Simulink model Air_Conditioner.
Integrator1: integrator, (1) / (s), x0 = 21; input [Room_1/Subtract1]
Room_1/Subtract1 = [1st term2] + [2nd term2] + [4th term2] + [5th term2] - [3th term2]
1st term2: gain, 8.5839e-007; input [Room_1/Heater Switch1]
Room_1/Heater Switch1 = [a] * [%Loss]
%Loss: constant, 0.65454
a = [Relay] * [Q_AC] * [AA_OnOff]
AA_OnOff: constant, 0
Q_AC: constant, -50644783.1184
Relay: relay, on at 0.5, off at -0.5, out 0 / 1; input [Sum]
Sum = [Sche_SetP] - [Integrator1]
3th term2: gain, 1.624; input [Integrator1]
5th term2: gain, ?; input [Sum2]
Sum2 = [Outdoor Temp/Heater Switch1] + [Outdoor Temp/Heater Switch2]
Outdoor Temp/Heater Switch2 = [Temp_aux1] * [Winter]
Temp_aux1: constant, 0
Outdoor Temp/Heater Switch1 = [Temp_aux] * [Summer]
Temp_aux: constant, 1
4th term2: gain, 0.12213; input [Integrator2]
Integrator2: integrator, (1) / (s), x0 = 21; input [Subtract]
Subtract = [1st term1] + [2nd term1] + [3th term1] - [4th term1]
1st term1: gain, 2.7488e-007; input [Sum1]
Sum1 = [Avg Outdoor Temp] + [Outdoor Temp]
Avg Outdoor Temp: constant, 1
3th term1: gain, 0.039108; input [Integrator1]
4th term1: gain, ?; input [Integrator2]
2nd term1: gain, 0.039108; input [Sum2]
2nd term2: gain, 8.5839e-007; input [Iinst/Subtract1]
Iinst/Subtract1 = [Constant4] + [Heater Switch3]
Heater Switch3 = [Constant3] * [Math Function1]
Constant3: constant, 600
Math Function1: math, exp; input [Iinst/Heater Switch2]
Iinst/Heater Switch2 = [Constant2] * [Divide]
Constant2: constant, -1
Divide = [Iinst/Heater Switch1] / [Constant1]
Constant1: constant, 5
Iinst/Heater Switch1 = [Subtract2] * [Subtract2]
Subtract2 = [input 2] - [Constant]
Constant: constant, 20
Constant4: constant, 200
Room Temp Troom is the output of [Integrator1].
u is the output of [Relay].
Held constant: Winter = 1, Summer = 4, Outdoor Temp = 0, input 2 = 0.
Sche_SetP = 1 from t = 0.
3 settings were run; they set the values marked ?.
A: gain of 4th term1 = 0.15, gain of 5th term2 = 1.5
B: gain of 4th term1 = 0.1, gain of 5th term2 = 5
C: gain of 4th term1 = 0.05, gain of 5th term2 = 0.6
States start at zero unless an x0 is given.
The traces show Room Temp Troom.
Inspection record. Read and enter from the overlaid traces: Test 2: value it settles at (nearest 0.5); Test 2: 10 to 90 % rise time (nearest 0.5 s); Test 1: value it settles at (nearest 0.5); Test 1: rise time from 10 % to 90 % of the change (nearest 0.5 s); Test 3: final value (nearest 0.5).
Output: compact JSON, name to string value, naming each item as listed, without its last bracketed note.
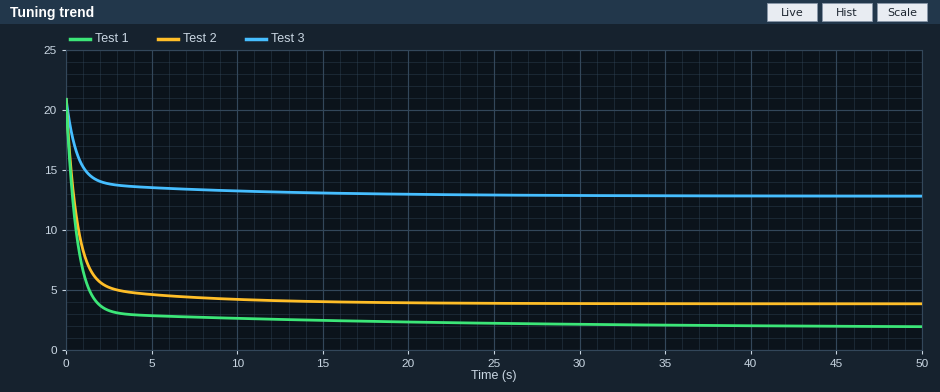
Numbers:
{"Test 2: value it settles at": "4.0", "Test 2: 10 to 90 % rise time": "2.0 s", "Test 1: value it settles at": "2.0", "Test 1: rise time from 10 % to 90 % of the change": "2.0 s", "Test 3: final value": "13.0"}
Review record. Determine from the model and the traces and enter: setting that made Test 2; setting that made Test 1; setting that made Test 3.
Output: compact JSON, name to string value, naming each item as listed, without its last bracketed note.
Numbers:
{"setting that made Test 2": "A", "setting that made Test 1": "C", "setting that made Test 3": "B"}
